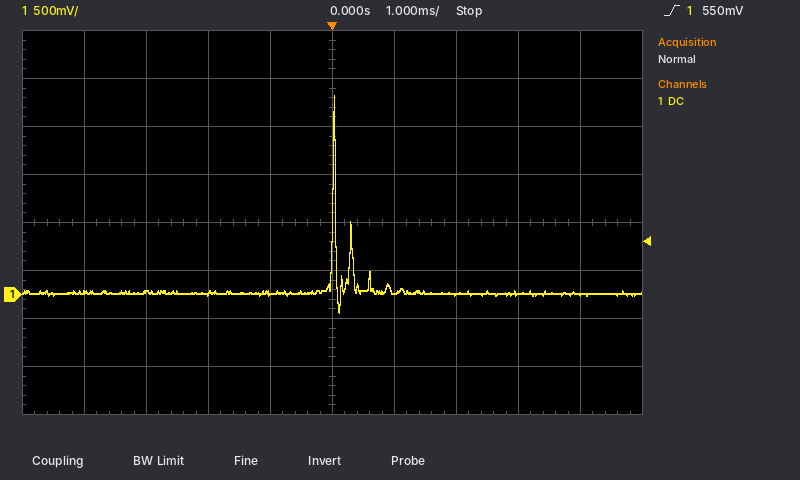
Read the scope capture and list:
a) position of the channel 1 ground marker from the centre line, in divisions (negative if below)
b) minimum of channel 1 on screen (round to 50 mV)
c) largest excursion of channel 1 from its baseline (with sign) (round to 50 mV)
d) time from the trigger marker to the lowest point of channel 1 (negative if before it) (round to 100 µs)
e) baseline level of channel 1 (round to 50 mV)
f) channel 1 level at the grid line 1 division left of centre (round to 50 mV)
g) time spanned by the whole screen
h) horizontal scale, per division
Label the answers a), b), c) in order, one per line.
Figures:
a) -1.5 div
b) -200 mV
c) +2.05 V
d) +100 µs
e) 0 mV
f) 0 mV
g) 10 ms
h) 1 ms
